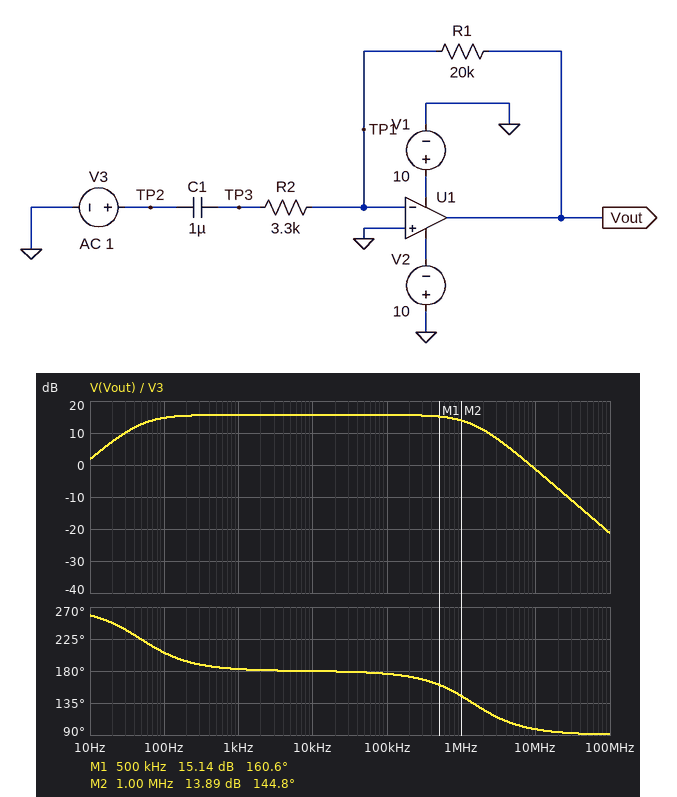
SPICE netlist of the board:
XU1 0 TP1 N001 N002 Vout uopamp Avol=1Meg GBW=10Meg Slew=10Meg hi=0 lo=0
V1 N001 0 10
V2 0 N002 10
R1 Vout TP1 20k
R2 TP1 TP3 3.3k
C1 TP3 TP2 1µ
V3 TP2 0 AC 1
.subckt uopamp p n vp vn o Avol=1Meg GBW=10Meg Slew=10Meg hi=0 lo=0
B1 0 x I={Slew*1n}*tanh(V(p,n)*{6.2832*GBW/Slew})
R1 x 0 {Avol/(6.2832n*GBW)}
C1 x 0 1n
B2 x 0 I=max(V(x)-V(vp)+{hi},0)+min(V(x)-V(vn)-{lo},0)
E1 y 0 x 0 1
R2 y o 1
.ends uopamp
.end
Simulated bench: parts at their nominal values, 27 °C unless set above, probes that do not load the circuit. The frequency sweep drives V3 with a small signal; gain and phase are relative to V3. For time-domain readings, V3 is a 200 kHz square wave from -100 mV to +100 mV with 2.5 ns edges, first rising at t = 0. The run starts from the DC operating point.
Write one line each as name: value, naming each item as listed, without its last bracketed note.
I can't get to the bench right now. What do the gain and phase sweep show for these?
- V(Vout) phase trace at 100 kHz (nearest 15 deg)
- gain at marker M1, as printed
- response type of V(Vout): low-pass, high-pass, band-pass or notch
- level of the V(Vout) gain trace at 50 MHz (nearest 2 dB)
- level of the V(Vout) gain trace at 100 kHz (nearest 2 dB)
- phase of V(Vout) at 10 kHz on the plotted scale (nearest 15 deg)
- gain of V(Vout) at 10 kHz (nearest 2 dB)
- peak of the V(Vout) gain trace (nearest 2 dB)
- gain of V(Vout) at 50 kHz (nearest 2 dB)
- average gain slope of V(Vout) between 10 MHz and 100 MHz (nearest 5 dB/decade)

V(Vout) phase trace at 100 kHz: 180 deg
gain at marker M1, as printed: 15.14 dB
response type of V(Vout): low-pass, high-pass, band-pass or notch: band-pass
level of the V(Vout) gain trace at 50 MHz: -16 dB
level of the V(Vout) gain trace at 100 kHz: 16 dB
phase of V(Vout) at 10 kHz on the plotted scale: 180 deg
gain of V(Vout) at 10 kHz: 16 dB
peak of the V(Vout) gain trace: 16 dB
gain of V(Vout) at 50 kHz: 16 dB
average gain slope of V(Vout) between 10 MHz and 100 MHz: -20 dB/decade
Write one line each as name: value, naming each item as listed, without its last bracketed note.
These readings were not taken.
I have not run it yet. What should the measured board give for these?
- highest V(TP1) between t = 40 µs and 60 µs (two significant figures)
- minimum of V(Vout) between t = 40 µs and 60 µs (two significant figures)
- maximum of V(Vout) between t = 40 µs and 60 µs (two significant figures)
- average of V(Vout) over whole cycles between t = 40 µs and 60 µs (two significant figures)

highest V(TP1) between t = 40 µs and 60 µs: 170 mV
minimum of V(Vout) between t = 40 µs and 60 µs: -1.2 V
maximum of V(Vout) between t = 40 µs and 60 µs: 11 mV
average of V(Vout) over whole cycles between t = 40 µs and 60 µs: -600 mV
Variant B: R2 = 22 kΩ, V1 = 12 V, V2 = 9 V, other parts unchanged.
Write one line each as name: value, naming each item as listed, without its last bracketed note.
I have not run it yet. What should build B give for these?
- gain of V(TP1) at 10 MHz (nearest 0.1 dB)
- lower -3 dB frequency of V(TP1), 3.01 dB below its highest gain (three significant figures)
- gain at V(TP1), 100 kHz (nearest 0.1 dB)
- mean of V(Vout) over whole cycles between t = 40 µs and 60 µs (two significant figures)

gain of V(TP1) at 10 MHz: -7.5 dB
lower -3 dB frequency of V(TP1), 3.01 dB below its highest gain: 5.24 MHz
gain at V(TP1), 100 kHz: -40.8 dB
mean of V(Vout) over whole cycles between t = 40 µs and 60 µs: -91 mV
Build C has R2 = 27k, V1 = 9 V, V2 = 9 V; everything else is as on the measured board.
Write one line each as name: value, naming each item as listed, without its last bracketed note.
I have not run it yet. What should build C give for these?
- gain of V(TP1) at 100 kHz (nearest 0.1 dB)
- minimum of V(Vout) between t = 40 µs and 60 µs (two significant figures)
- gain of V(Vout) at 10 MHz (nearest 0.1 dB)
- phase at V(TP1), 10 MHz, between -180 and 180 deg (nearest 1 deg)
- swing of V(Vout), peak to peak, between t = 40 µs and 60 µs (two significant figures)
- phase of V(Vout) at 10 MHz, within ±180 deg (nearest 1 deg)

gain of V(TP1) at 100 kHz: -42.6 dB
minimum of V(Vout) between t = 40 µs and 60 µs: -150 mV
gain of V(Vout) at 10 MHz: -8.7 dB
phase at V(TP1), 10 MHz, between -180 and 180 deg: 30 deg
swing of V(Vout), peak to peak, between t = 40 µs and 60 µs: 150 mV
phase of V(Vout) at 10 MHz, within ±180 deg: 120 deg
